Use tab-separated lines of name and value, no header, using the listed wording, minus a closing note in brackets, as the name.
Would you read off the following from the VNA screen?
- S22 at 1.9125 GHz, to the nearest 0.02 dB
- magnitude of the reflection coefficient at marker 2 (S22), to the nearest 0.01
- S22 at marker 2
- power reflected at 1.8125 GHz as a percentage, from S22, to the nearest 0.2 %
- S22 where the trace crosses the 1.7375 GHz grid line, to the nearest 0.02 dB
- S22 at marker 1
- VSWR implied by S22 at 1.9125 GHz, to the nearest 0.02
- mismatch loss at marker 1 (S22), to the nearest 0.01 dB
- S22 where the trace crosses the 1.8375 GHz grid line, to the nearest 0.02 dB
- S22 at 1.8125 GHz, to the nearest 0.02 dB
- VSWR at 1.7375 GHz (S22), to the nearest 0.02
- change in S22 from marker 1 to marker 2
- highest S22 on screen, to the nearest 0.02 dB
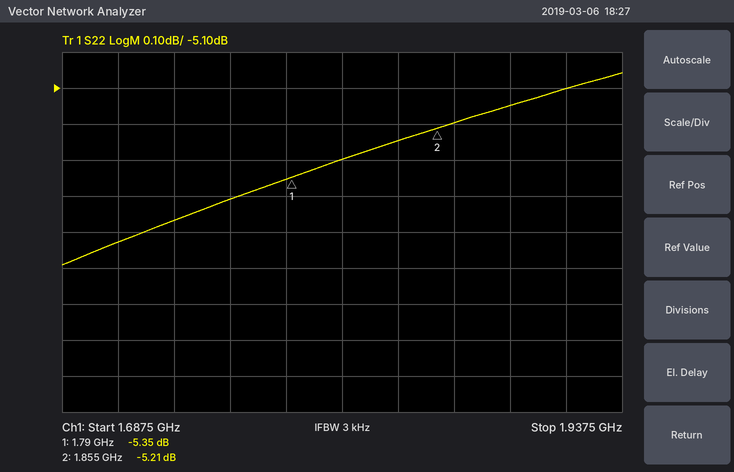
S22 at 1.9125 GHz, to the nearest 0.02 dB	-5.10 dB
magnitude of the reflection coefficient at marker 2 (S22), to the nearest 0.01	0.55
S22 at marker 2	-5.21 dB
power reflected at 1.8125 GHz as a percentage, from S22, to the nearest 0.2 %	29.6 %
S22 where the trace crosses the 1.7375 GHz grid line, to the nearest 0.02 dB	-5.46 dB
S22 at marker 1	-5.35 dB
VSWR implied by S22 at 1.9125 GHz, to the nearest 0.02	3.50
mismatch loss at marker 1 (S22), to the nearest 0.01 dB	1.50 dB
S22 where the trace crosses the 1.8375 GHz grid line, to the nearest 0.02 dB	-5.24 dB
S22 at 1.8125 GHz, to the nearest 0.02 dB	-5.30 dB
VSWR at 1.7375 GHz (S22), to the nearest 0.02	3.28
change in S22 from marker 1 to marker 2	0.14 dB
highest S22 on screen, to the nearest 0.02 dB	-5.06 dB
